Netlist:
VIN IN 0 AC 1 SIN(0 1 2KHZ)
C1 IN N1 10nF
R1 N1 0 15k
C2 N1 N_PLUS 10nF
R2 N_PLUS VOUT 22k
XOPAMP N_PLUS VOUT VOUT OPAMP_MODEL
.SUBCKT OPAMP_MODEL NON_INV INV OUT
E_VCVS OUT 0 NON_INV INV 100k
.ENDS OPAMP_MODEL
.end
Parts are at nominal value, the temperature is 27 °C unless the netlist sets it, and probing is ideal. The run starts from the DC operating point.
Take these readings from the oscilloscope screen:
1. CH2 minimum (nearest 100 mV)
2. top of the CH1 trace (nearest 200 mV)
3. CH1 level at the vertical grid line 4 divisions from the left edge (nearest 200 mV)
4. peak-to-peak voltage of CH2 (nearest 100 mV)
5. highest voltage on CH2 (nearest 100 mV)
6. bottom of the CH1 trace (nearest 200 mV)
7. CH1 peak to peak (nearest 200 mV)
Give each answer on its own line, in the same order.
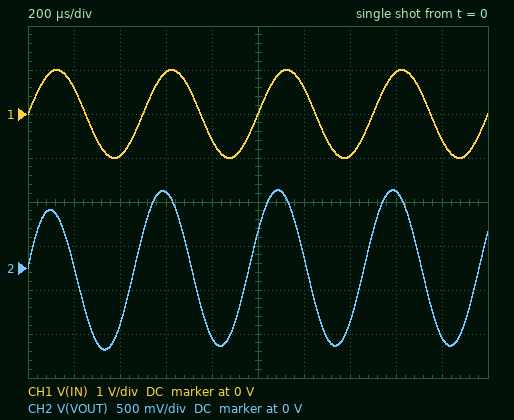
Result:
-900 mV
1.0 V
-600 mV
1.8 V
900 mV
-1.0 V
2.0 V
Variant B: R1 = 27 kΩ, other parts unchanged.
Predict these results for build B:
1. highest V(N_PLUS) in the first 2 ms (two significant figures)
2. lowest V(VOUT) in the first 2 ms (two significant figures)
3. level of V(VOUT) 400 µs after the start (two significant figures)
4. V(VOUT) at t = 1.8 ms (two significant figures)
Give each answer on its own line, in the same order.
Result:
960 mV
-1.0 V
-850 mV
-760 mV
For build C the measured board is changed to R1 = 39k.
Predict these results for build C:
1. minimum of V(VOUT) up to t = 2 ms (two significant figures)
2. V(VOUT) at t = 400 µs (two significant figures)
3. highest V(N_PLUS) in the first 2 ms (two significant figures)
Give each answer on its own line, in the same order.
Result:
-1.1 V
-920 mV
980 mV
